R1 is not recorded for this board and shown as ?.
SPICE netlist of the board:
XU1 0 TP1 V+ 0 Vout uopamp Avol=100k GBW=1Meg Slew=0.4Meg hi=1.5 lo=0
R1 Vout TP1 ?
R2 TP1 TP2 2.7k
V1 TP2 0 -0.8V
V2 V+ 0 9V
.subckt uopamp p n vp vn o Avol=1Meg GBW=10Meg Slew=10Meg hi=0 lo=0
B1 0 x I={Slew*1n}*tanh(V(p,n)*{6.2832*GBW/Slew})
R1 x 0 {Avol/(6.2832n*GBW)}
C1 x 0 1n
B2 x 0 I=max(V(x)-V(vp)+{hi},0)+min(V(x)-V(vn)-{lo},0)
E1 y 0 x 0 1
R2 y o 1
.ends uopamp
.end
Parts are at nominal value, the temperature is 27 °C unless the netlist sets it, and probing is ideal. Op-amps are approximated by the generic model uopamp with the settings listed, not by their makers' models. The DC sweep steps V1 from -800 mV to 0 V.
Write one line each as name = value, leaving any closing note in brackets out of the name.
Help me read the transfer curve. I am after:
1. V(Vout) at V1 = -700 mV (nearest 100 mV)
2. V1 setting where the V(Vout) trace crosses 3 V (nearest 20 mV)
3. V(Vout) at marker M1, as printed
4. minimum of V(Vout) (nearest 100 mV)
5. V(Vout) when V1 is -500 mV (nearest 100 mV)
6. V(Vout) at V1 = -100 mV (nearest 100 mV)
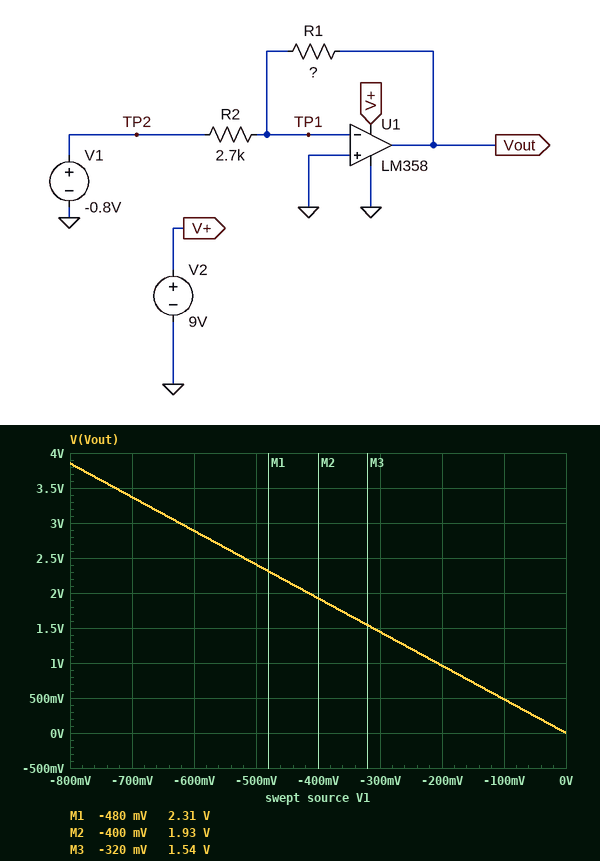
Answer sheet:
V(Vout) at V1 = -700 mV = 3.4 V
V1 setting where the V(Vout) trace crosses 3 V = -620 mV
V(Vout) at marker M1, as printed = 2.31 V
minimum of V(Vout) = 0 V
V(Vout) when V1 is -500 mV = 2.4 V
V(Vout) at V1 = -100 mV = 500 mV
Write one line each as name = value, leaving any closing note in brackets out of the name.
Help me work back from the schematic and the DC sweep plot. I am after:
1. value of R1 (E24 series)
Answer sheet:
value of R1 = 13 kΩ
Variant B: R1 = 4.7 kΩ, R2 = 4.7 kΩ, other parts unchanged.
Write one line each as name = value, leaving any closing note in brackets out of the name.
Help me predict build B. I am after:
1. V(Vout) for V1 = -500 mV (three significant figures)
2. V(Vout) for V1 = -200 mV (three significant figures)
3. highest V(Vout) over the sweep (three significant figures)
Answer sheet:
V(Vout) for V1 = -500 mV = 500 mV
V(Vout) for V1 = -200 mV = 200 mV
highest V(Vout) over the sweep = 800 mV
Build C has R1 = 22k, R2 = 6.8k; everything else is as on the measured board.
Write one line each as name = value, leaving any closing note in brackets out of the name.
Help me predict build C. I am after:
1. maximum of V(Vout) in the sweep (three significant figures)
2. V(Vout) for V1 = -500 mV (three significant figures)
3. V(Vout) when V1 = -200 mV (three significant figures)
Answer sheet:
maximum of V(Vout) in the sweep = 2.59 V
V(Vout) for V1 = -500 mV = 1.62 V
V(Vout) when V1 = -200 mV = 647 mV
